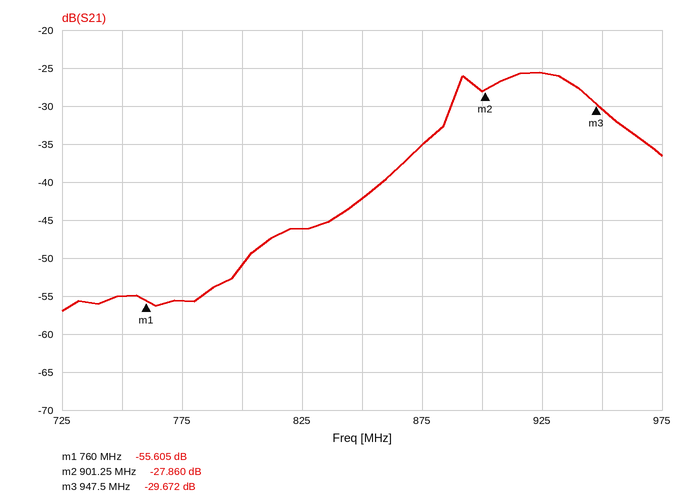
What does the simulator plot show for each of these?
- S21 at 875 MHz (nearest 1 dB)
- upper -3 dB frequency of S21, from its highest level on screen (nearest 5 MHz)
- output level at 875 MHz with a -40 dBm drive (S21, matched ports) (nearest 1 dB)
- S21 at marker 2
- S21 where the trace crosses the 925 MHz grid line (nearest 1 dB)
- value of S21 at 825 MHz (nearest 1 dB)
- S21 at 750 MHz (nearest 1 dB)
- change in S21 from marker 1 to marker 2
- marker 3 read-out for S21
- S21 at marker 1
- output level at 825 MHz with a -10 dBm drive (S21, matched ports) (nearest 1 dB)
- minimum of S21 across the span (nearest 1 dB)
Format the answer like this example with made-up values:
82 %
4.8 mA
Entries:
-35 dB
945 MHz
-75 dBm
-27.860 dB
-26 dB
-46 dB
-55 dB
27.745 dB
-29.672 dB
-55.605 dB
-56 dBm
-57 dB
